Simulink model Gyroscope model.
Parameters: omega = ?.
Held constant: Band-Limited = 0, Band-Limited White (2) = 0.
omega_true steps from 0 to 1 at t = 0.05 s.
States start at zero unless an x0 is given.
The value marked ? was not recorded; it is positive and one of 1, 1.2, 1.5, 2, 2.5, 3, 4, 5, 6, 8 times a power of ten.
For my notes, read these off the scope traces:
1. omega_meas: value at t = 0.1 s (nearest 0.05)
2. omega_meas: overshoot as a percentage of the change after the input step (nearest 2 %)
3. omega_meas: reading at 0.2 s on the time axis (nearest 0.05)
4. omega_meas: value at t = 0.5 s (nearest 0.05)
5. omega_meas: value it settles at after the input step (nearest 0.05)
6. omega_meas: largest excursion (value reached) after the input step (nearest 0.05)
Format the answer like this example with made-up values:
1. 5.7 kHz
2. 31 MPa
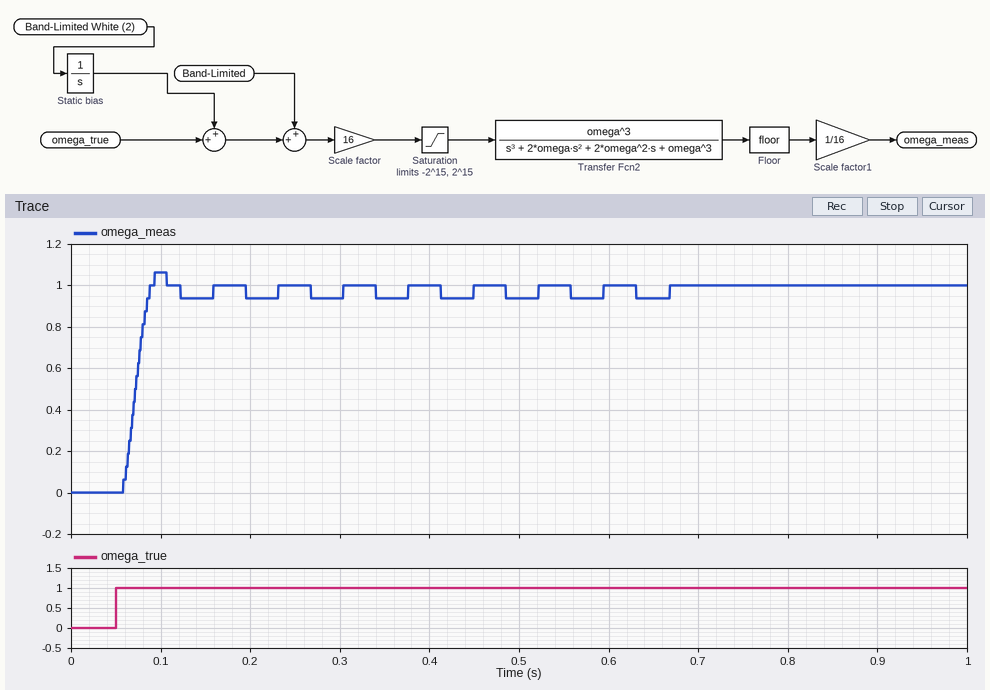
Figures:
1. 1.05
2. 6 %
3. 0.95
4. 0.95
5. 1.00
6. 1.05
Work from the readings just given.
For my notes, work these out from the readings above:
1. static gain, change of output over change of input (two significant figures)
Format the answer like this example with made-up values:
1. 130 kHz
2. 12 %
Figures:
1. 1.0
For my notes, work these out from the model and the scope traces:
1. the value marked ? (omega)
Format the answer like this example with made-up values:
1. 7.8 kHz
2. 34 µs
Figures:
1. 100
